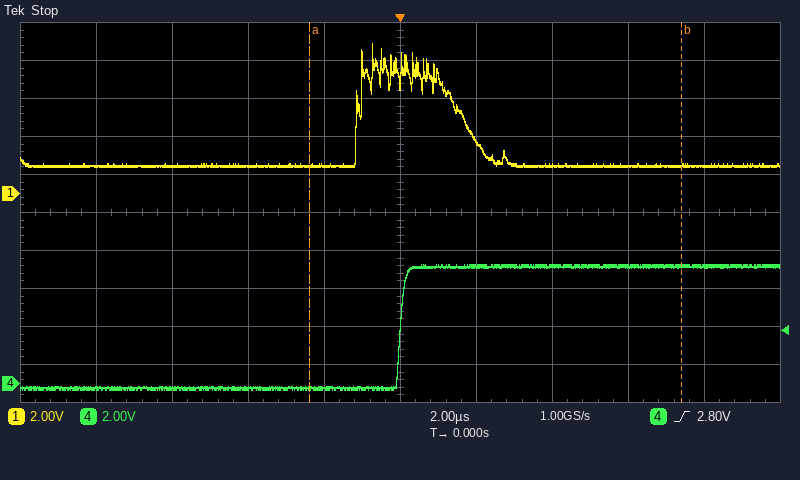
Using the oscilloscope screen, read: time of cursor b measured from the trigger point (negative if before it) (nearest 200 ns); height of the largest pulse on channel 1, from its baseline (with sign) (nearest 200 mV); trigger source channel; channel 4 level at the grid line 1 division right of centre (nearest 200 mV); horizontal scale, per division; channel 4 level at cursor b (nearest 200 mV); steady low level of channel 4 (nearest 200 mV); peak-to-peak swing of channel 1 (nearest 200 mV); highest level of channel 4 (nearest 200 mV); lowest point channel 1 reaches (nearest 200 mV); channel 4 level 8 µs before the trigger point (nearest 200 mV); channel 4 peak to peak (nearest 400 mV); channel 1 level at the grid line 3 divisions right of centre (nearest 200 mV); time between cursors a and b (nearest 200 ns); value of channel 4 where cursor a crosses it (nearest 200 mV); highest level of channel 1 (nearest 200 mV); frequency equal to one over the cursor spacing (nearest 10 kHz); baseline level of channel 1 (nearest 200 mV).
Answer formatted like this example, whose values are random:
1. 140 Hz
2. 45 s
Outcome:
1. +7.4 µs
2. +6.4 V
3. channel 4
4. 6.2 V
5. 2 µs
6. 6.2 V
7. -200 mV
8. 6.4 V
9. 6.2 V
10. 1.4 V
11. -200 mV
12. 6.4 V
13. 1.4 V
14. 9.8 µs
15. -200 mV
16. 7.8 V
17. 100 kHz
18. 1.4 V
